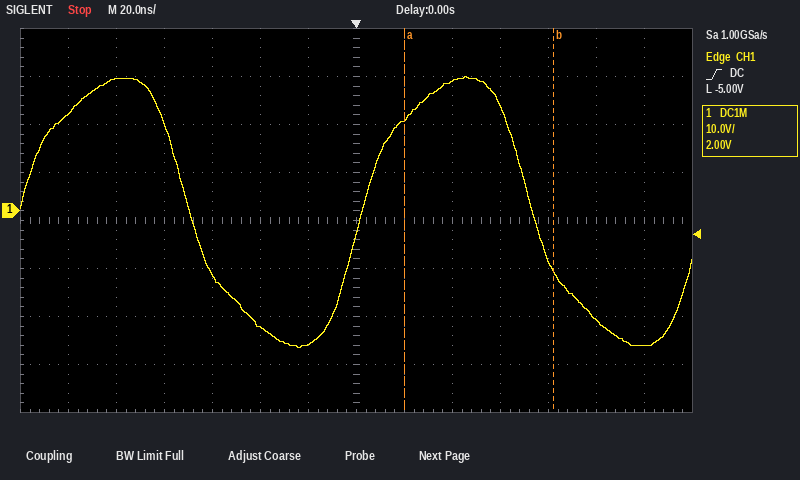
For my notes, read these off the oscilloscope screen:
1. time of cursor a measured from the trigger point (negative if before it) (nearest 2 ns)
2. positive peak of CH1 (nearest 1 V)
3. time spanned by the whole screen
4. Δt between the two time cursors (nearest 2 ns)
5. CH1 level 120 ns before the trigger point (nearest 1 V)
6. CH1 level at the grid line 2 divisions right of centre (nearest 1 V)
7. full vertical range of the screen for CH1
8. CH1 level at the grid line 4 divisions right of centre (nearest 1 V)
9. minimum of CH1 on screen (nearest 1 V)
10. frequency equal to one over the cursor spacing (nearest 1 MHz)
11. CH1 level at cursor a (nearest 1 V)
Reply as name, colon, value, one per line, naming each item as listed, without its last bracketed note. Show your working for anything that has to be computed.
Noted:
time of cursor a measured from the trigger point (negative if before it): +20 ns
positive peak of CH1: 28 V
time spanned by the whole screen: 280 ns
Δt between the two time cursors: 62 ns
CH1 level 120 ns before the trigger point: 20 V
CH1 level at the grid line 2 divisions right of centre: 27 V
full vertical range of the screen for CH1: 80 V
CH1 level at the grid line 4 divisions right of centre: -10 V
minimum of CH1 on screen: -28 V
frequency equal to one over the cursor spacing: 1 / 62 ns ≈ 16 MHz
CH1 level at cursor a: 19 V
